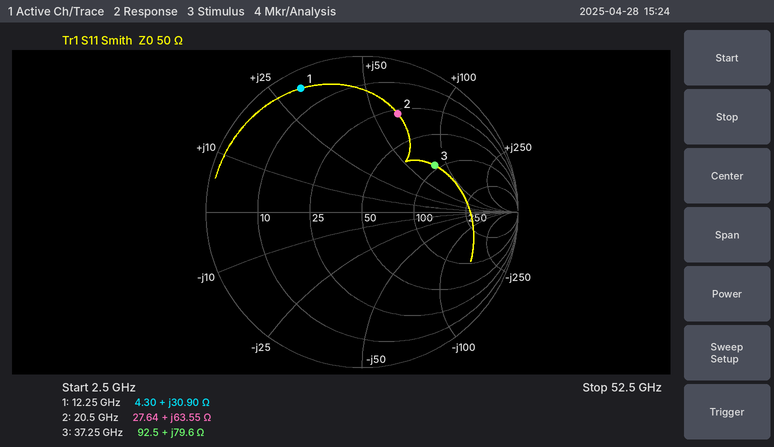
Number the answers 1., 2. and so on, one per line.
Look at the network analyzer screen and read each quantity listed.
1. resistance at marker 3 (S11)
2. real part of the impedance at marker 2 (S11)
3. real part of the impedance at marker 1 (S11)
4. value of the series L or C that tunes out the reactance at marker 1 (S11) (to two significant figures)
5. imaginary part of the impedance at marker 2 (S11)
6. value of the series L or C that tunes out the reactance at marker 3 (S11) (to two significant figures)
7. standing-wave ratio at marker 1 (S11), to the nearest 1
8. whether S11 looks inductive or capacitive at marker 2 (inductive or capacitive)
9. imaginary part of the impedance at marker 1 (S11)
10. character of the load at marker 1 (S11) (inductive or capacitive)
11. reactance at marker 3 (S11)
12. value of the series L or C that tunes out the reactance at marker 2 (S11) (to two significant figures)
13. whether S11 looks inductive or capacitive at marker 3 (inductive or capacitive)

1. 92.5 Ω
2. 27.64 Ω
3. 4.30 Ω
4. 420 fF
5. +63.55 Ω
6. 54 fF
7. 16
8. inductive
9. +30.90 Ω
10. inductive
11. +79.6 Ω
12. 120 fF
13. inductive
